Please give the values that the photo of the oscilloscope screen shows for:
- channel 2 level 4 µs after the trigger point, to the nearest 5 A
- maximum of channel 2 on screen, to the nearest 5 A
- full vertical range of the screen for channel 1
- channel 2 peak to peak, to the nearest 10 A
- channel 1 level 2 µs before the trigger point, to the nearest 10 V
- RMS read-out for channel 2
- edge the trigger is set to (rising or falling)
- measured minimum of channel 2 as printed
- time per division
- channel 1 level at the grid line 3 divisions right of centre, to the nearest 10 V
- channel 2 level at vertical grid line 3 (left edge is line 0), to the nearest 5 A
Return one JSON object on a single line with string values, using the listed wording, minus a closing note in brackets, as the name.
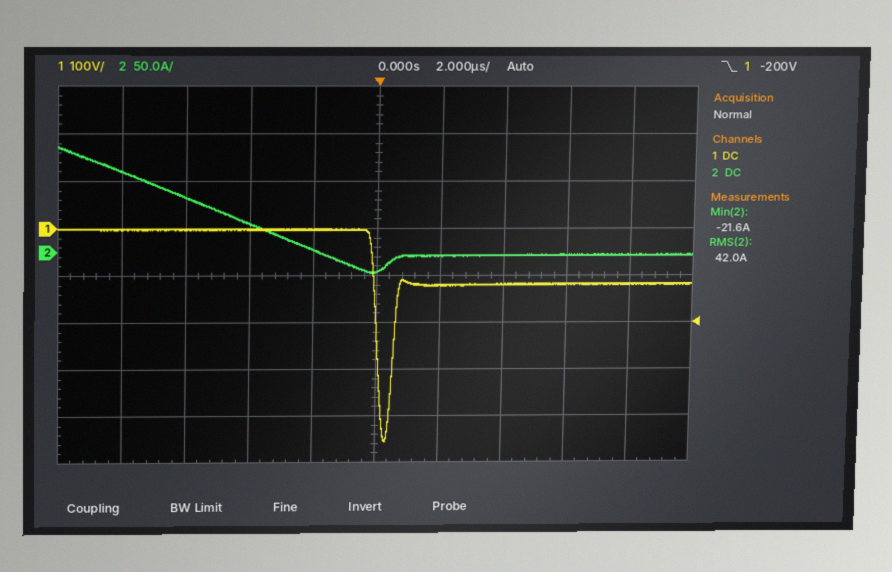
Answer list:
{"channel 2 level 4 µs after the trigger point, to the nearest 5 A": "-5 A", "maximum of channel 2 on screen, to the nearest 5 A": "110 A", "full vertical range of the screen for channel 1": "800 V", "channel 2 peak to peak, to the nearest 10 A": "130 A", "channel 1 level 2 µs before the trigger point, to the nearest 10 V": "0 V", "RMS read-out for channel 2": "42.0 A", "edge the trigger is set to": "falling", "measured minimum of channel 2 as printed": "-21.6 A", "time per division": "2 µs", "channel 1 level at the grid line 3 divisions right of centre, to the nearest 10 V": "-120 V", "channel 2 level at vertical grid line 3 (left edge is line 0), to the nearest 5 A": "30 A"}
